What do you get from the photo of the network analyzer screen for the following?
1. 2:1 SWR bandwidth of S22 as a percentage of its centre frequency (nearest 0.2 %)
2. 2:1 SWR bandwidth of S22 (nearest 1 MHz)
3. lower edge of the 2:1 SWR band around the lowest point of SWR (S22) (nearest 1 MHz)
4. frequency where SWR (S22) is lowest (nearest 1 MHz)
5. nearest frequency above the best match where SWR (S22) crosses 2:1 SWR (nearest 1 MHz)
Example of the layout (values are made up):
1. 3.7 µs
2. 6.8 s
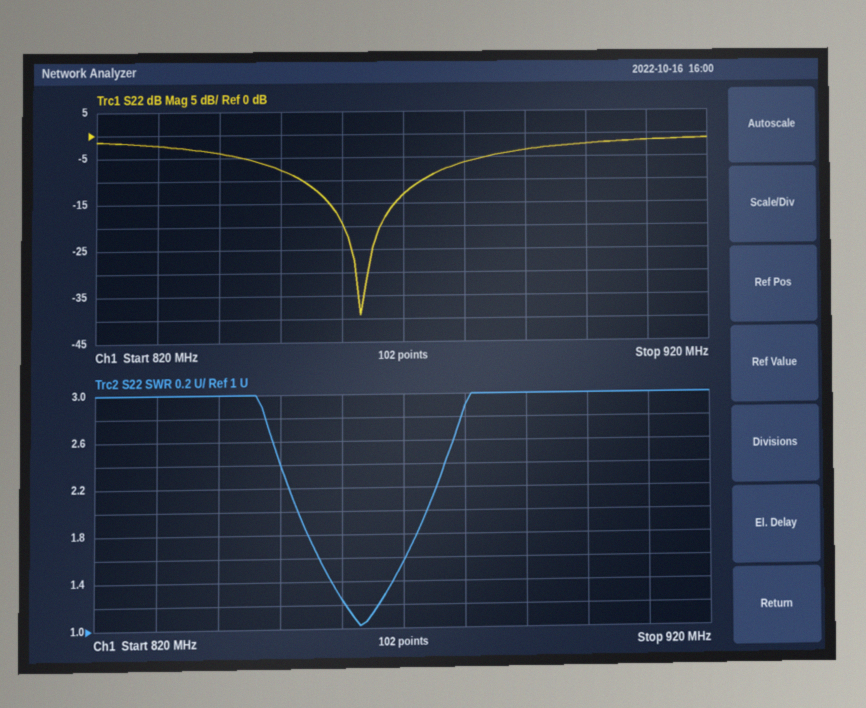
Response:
1. 2.4 %
2. 21 MHz
3. 853 MHz
4. 863 MHz
5. 874 MHz
